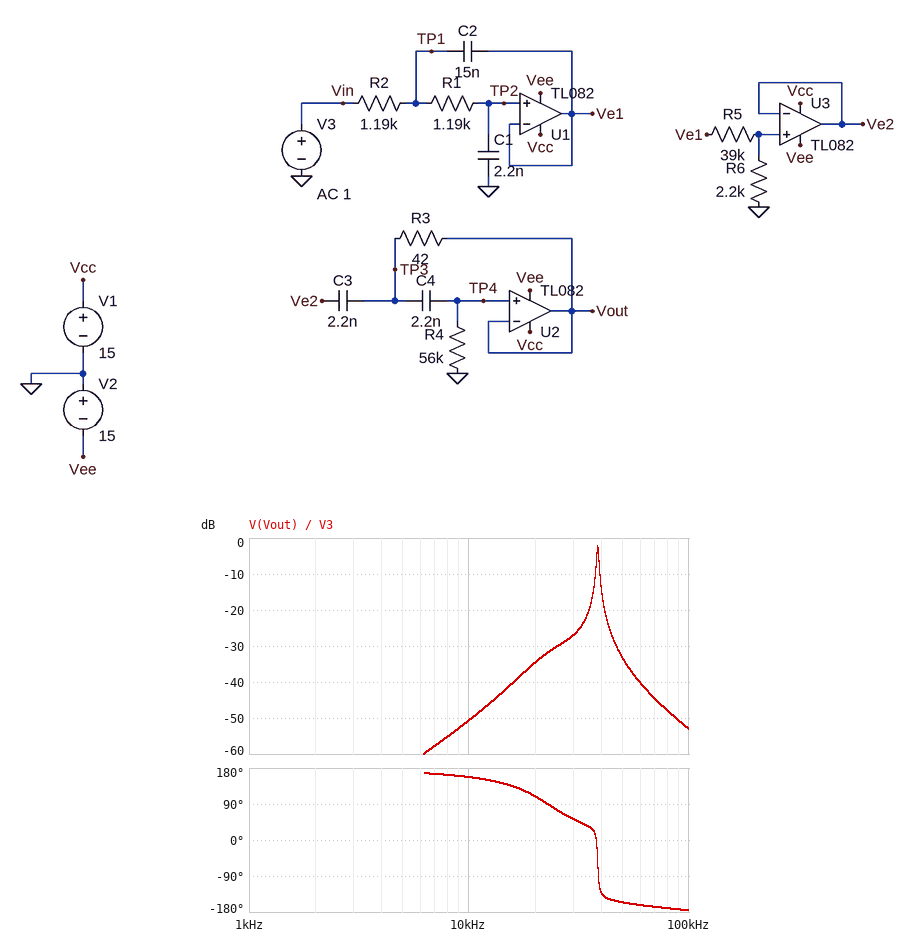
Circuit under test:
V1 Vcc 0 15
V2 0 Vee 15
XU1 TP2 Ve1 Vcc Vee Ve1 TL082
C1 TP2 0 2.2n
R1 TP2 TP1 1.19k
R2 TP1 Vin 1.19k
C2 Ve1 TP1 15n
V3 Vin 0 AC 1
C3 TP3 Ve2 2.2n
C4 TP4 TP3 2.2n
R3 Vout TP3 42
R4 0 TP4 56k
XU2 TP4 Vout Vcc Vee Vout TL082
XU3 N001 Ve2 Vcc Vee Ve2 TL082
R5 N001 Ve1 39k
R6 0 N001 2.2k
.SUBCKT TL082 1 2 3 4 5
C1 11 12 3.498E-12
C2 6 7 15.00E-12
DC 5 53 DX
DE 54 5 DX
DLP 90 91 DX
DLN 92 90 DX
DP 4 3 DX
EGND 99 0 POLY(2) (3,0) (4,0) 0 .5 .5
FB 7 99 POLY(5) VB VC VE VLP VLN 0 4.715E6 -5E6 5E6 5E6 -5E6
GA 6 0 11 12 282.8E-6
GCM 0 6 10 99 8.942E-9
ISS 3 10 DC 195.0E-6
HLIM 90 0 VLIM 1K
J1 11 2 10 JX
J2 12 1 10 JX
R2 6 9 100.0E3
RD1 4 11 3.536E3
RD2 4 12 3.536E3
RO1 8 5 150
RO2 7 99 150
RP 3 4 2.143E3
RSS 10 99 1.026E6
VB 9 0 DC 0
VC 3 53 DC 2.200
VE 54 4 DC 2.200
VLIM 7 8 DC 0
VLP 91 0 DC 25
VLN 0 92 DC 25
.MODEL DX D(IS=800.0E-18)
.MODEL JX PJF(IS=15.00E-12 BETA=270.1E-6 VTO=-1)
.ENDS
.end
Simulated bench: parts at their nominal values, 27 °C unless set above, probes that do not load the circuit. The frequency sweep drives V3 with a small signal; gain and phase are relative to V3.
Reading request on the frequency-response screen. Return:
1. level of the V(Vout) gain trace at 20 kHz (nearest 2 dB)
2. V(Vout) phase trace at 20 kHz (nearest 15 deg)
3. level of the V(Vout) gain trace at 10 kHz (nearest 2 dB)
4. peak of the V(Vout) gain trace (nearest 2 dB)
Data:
-34 dB
105 deg
-50 dB
-2 dB
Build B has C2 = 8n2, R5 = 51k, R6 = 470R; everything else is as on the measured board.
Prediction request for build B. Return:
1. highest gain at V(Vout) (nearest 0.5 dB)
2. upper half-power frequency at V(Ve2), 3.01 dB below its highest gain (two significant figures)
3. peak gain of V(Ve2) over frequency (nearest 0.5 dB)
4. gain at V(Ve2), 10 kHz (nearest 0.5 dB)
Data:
-13.5 dB
36 kHz
-39.5 dB
-40.5 dB
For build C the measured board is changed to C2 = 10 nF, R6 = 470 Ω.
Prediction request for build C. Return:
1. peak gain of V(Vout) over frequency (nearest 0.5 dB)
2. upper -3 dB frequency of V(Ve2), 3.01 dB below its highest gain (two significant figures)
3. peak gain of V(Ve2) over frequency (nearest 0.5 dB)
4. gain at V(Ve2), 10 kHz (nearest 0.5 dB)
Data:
-12.0 dB
33 kHz
-37.0 dB
-38.0 dB
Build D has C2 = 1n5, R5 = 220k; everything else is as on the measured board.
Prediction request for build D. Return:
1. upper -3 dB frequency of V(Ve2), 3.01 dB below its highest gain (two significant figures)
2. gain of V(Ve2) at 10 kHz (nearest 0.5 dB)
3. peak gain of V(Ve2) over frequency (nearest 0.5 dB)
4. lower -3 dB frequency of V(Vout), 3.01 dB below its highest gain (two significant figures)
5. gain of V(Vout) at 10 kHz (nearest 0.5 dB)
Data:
37 kHz
-40.5 dB
-40.0 dB
38 kHz
-66.5 dB
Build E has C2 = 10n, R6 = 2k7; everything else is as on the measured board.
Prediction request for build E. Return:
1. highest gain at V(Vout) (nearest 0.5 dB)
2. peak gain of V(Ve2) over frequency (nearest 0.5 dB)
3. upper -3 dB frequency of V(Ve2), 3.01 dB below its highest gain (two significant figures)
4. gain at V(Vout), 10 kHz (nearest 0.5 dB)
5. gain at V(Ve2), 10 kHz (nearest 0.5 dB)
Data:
2.5 dB
-22.0 dB
33 kHz
-49.5 dB
-23.0 dB
